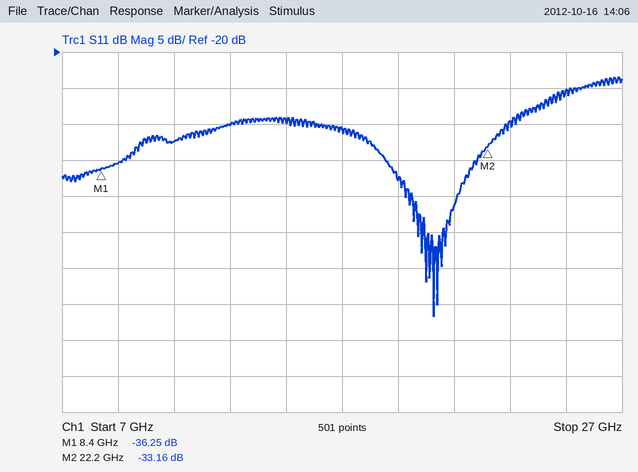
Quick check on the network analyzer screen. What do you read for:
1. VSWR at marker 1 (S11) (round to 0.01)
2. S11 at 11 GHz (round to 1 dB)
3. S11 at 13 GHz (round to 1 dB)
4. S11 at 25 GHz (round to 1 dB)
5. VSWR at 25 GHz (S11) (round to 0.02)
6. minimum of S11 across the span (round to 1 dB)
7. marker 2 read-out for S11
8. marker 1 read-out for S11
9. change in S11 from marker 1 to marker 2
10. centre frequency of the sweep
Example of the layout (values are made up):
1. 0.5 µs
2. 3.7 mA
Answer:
1. 1.03
2. -32 dB
3. -30 dB
4. -25 dB
5. 1.12
6. -57 dB
7. -33.16 dB
8. -36.25 dB
9. 3.09 dB
10. 17 GHz
